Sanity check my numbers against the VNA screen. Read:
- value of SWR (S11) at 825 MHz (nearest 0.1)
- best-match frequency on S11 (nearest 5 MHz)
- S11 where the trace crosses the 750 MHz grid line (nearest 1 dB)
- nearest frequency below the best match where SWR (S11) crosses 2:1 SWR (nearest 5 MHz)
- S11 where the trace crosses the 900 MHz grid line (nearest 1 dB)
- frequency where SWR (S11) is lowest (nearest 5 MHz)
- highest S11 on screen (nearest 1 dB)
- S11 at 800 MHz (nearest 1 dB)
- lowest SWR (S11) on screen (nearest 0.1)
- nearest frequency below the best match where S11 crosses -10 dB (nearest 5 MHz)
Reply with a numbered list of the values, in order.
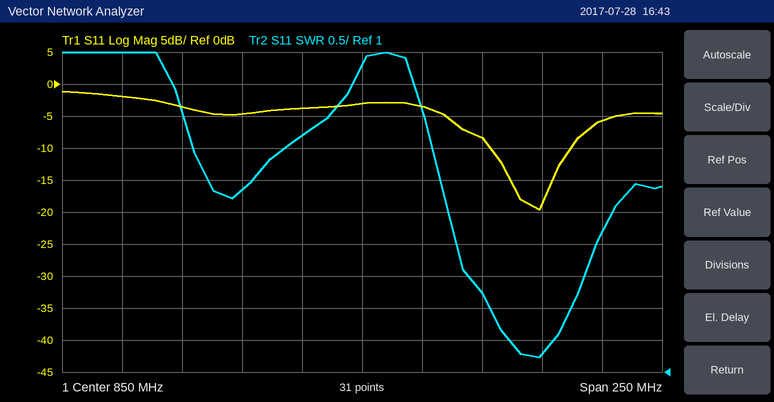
1. 4.7
2. 925 MHz
3. -2 dB
4. 905 MHz
5. -8 dB
6. 925 MHz
7. -1 dB
8. -5 dB
9. 1.2
10. 905 MHz
